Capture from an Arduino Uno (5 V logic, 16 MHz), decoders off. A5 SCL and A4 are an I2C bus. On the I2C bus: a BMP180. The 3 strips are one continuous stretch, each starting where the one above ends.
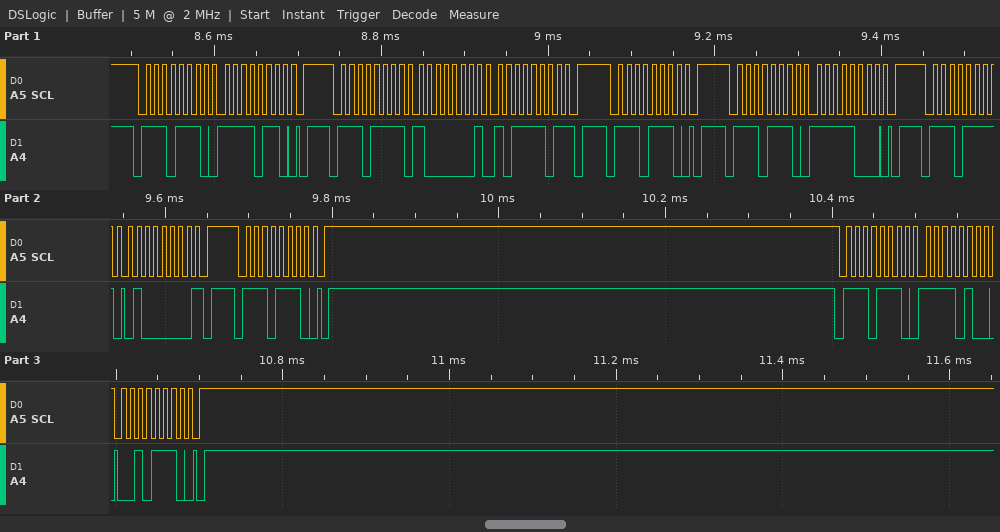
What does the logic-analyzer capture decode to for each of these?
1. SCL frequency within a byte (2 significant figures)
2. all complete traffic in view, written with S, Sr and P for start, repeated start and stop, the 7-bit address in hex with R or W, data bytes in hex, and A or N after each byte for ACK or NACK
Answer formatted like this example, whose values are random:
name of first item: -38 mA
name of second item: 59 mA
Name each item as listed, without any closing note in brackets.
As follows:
SCL frequency within a byte: 100 kHz
all complete traffic in view, written with S, Sr and P for start, repeated start and stop, the 7-bit address in hex with R or W, data bytes in hex, and A or N after each byte for ACK or NACK: S 77W A F6 A P S 77R A 81 A BD N P S 77W A P S 77W A F8 A P S 77R A 40 N P S 77W A P S 77W A F4 A 2E A P
